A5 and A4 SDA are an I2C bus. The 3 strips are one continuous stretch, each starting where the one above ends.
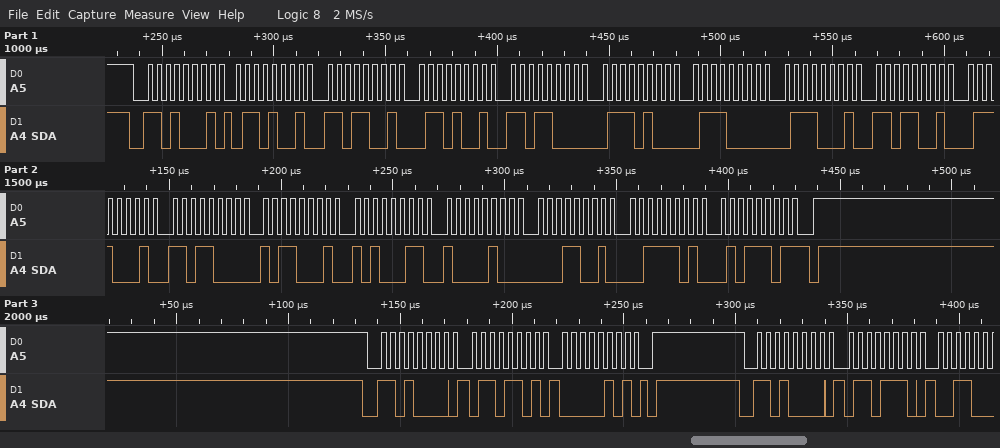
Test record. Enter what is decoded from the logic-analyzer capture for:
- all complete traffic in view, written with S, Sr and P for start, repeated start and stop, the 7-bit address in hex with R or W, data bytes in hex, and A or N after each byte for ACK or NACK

S 68R A 69 A D9 A 69 A D8 A 74 A 70 A 71 A D9 A 71 A D8 A B1 A A3 A 84 A 19 A 3D A 5D N P S 68W A 6D A 05 A P S 68W A 6E A
